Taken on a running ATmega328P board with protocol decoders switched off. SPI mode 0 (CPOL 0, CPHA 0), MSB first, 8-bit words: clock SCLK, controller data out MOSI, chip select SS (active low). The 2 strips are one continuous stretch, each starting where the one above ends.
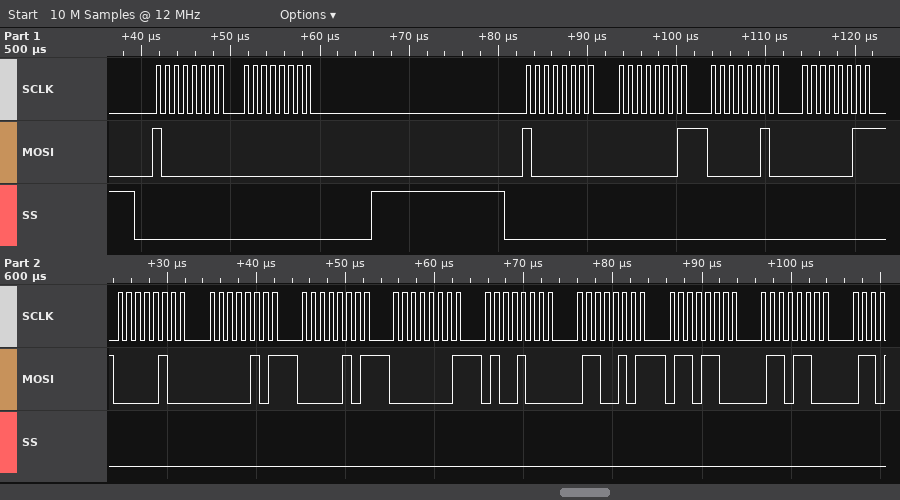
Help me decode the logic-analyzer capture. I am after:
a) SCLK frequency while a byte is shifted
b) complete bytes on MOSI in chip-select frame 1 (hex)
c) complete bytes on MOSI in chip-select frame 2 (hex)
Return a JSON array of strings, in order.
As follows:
["1 MHz", "80 00", "80 01 02 03 04 05 05 01 48 65 6C 6C"]
